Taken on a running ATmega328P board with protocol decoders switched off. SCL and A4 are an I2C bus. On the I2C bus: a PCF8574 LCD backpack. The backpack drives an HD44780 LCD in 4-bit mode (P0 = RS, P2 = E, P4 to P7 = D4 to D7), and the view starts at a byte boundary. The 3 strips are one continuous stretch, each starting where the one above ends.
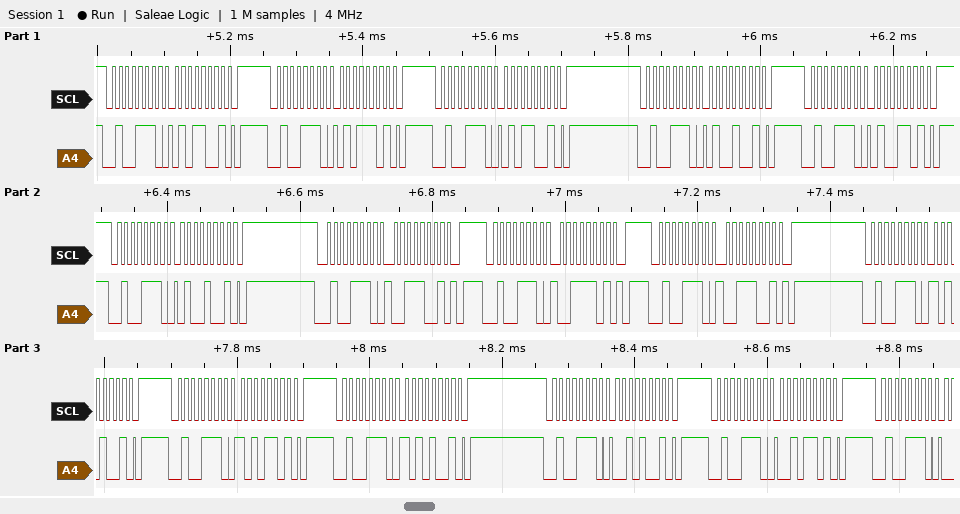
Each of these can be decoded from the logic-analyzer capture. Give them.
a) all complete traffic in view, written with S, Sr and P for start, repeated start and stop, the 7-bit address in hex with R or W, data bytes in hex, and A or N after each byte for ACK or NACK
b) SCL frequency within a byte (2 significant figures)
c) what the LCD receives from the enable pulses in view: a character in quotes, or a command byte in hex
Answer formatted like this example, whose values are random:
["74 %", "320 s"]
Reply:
["S 27W A 59 A P S 27W A 5D A P S 27W A 59 A P S 27W A 49 A P S 27W A 4D A P S 27W A 49 A P S 27W A 39 A P S 27W A 3D A P S 27W A 39 A P S 27W A A9 A P S 27W A AD A P S 27W A A9 A P S 27W A 29 A P S 27W A 2D A P S 27W A", "100 kHz", "'T' ':'"]
